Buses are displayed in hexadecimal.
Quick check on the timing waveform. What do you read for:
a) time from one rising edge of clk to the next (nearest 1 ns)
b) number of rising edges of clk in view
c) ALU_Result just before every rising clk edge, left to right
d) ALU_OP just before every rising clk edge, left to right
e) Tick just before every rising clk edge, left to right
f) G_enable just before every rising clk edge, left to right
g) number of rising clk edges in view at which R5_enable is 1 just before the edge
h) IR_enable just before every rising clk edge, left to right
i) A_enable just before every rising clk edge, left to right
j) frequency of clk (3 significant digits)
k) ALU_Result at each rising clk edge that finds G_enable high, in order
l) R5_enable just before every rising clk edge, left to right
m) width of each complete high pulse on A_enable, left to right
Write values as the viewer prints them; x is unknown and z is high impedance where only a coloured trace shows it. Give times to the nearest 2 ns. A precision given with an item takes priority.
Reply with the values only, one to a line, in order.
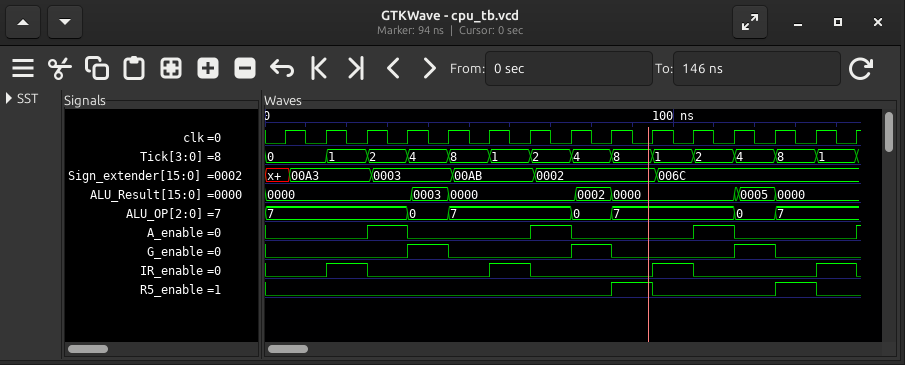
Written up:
10 ns
15
0000, 0000, 0000, 0000, 0003, 0000, 0000, 0000, 0002, 0000, 0000, 0000, 0005, 0000, 0000
7, 7, 7, 7, 0, 7, 7, 7, 0, 7, 7, 7, 0, 7, 7
0, 0, 1, 2, 4, 8, 1, 2, 4, 8, 1, 2, 4, 8, 1
0 0 0 0 1 0 0 0 1 0 0 0 1 0 0
2
0 0 1 0 0 0 1 0 0 0 1 0 0 0 1
0 0 0 1 0 0 0 1 0 0 0 1 0 0 0
100 MHz
0003, 0002, 0005
0 0 0 0 0 0 0 0 0 1 0 0 0 1 0
10 ns, 10 ns, 10 ns
